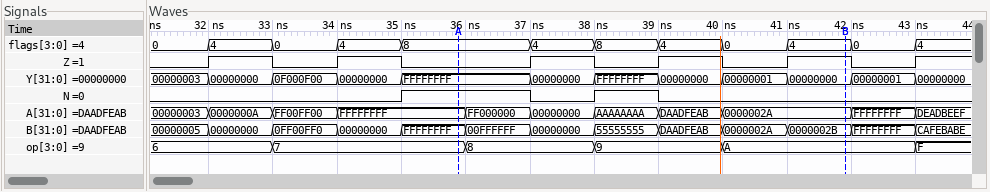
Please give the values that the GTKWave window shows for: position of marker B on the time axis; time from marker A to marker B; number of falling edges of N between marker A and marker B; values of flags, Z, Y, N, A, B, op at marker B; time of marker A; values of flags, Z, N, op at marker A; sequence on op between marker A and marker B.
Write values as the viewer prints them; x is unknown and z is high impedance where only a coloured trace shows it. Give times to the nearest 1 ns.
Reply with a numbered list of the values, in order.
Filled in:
1. 42 ns
2. 6 ns
3. 2
4. flags=4, Z=1, Y=00000000, N=0, A=0000002A, B=0000002B, op=A
5. 36 ns
6. flags=8, Z=0, N=1, op=7
7. 7, 8, 9, A
